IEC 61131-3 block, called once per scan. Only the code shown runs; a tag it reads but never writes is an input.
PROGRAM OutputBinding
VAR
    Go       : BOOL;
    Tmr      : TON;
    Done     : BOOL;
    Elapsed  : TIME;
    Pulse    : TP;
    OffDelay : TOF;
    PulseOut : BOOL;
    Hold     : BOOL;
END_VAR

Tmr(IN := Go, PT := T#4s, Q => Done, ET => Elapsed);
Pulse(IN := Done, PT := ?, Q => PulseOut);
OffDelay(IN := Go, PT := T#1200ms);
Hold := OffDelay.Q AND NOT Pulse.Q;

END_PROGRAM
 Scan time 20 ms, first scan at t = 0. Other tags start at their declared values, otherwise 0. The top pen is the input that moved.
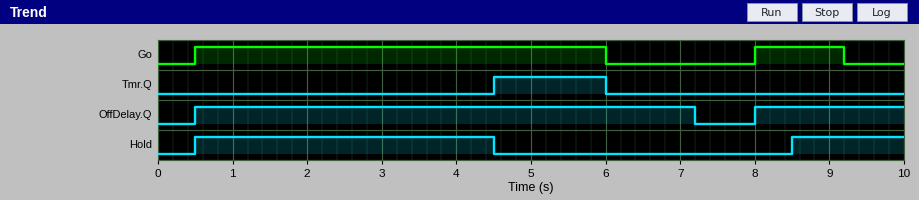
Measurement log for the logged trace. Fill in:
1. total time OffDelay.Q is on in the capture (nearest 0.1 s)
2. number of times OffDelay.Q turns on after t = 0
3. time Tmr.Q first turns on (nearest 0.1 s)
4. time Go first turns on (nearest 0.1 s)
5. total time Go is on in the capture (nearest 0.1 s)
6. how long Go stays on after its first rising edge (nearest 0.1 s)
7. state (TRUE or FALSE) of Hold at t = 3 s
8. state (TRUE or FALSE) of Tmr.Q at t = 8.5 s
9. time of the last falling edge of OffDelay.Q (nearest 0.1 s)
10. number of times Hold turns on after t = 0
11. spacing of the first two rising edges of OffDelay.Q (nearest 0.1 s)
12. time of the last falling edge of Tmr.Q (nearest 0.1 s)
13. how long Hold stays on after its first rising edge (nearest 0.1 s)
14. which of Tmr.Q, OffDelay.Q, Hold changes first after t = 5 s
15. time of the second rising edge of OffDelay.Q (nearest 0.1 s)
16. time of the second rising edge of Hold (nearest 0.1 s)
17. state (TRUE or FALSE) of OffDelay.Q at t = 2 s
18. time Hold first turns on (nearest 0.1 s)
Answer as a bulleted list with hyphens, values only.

- 8.7 s
- 2
- 4.5 s
- 0.5 s
- 6.7 s
- 5.5 s
- TRUE
- FALSE
- 7.2 s
- 2
- 7.5 s
- 6.0 s
- 4.0 s
- Tmr.Q
- 8.0 s
- 8.5 s
- TRUE
- 0.5 s
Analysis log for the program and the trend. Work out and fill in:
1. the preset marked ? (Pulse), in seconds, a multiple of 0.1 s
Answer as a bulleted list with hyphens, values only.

- 4.0 s
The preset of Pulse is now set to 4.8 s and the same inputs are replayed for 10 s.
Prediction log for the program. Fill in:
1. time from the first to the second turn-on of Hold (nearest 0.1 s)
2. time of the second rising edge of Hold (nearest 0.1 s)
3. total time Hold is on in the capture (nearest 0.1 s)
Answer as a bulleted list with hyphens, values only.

- 8.8 s
- 9.3 s
- 4.7 s
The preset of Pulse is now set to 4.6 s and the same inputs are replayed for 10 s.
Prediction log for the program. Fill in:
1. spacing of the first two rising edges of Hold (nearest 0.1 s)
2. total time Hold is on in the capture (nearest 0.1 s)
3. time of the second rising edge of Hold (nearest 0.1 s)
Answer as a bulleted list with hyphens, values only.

- 8.6 s
- 4.9 s
- 9.1 s
